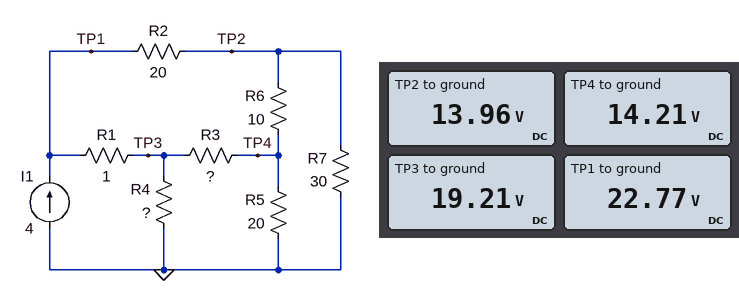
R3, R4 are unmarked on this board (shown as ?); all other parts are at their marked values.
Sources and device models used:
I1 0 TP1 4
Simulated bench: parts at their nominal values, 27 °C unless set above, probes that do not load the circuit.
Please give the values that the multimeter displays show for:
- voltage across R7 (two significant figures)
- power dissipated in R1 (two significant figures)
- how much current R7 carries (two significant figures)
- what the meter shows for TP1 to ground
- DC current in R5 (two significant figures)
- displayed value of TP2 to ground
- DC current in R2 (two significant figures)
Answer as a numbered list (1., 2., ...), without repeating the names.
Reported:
1. 14 V
2. 13 W
3. 470 mA
4. 22.77 V
5. 710 mA
6. 13.96 V
7. 440 mA
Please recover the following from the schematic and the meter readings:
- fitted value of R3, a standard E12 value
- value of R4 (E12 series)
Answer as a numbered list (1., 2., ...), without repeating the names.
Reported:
1. 6.8 Ω
2. 6.8 Ω
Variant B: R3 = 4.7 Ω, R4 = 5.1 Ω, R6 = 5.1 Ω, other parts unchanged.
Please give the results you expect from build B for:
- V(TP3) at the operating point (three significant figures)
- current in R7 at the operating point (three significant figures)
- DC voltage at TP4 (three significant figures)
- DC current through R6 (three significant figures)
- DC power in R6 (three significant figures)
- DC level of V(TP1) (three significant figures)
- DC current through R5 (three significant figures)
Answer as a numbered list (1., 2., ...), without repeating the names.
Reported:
1. 15.3 V
2. 398 mA
3. 12.2 V
4. 48.4 mA
5. 11.9 mW
6. 18.9 V
7. 609 mA
